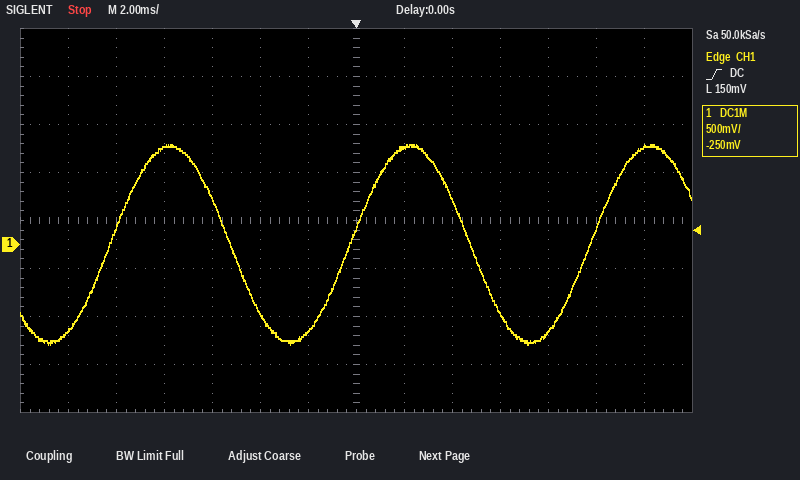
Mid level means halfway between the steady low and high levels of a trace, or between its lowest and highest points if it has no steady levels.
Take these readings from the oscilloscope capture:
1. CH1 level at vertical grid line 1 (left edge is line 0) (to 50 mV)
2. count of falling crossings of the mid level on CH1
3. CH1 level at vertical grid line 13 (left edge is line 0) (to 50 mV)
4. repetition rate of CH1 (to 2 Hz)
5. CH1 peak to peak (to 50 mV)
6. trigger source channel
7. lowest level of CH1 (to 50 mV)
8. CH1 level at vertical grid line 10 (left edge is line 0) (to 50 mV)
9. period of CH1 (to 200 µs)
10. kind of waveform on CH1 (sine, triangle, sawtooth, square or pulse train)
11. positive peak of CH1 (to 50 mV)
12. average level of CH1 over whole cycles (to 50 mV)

-900 mV
2
1.00 V
100 Hz
2.10 V
CH1
-1.05 V
-700 mV
10.0 ms
sine
1.05 V
0 mV
